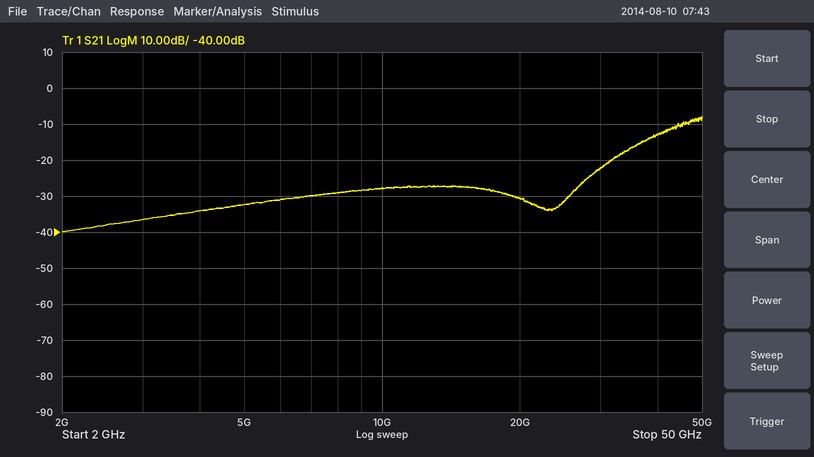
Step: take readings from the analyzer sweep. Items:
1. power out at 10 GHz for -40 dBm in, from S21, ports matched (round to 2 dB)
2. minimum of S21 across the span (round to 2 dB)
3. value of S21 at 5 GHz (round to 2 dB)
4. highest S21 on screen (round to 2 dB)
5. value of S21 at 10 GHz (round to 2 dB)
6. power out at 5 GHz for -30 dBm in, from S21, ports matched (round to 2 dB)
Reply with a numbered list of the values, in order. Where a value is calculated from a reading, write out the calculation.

1. -40 dBm + (-28 dB) = -68 dBm
2. -40 dB
3. -32 dB
4. -8 dB
5. -28 dB
6. -30 dBm + (-32 dB) = -62 dBm
